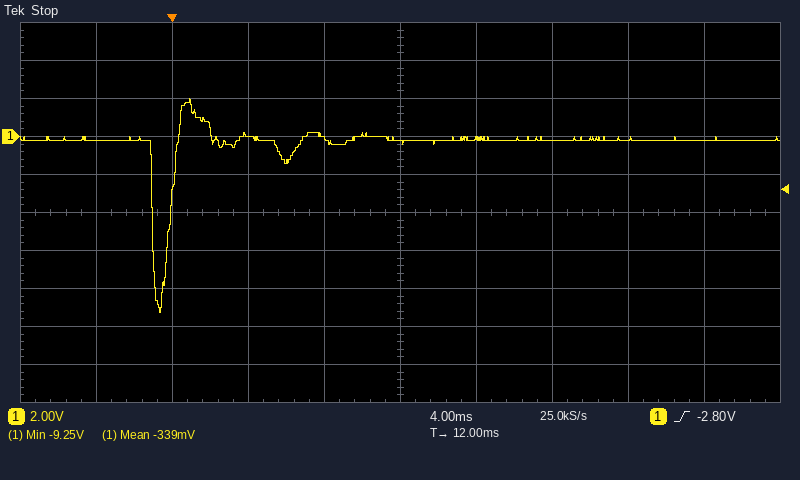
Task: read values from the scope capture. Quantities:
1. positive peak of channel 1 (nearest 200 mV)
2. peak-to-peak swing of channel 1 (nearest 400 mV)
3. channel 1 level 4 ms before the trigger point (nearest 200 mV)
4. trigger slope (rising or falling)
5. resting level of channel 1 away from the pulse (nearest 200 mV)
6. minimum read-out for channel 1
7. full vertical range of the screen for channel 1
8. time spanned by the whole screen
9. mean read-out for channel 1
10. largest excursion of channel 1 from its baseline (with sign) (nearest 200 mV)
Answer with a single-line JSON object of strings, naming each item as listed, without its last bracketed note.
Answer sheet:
{"positive peak of channel 1": "2.0 V", "peak-to-peak swing of channel 1": "11.2 V", "channel 1 level 4 ms before the trigger point": "-200 mV", "trigger slope": "rising", "resting level of channel 1 away from the pulse": "-200 mV", "minimum read-out for channel 1": "-9.25 V", "full vertical range of the screen for channel 1": "20 V", "time spanned by the whole screen": "40 ms", "mean read-out for channel 1": "-339 mV", "largest excursion of channel 1 from its baseline (with sign)": "-9.0 V"}
